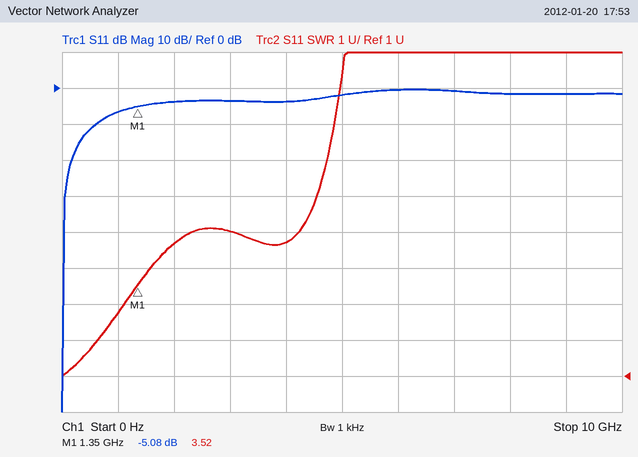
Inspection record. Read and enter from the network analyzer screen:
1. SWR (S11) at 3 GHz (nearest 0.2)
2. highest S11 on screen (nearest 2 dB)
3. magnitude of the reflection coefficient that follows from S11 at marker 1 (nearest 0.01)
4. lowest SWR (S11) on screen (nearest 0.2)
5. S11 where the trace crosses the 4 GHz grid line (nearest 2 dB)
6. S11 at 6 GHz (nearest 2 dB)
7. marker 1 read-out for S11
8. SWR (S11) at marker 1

5.0
0 dB
0.56
1.0
-4 dB
0 dB
-5.08 dB
3.52
